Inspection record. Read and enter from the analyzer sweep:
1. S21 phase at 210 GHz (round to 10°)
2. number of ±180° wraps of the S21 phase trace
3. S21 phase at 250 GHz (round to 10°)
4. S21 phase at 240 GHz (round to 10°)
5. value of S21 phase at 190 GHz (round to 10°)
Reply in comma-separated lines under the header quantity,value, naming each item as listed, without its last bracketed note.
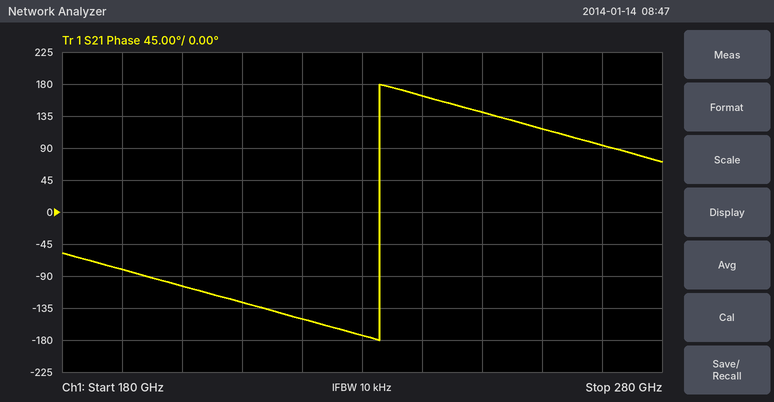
quantity,value
S21 phase at 210 GHz,-130°
number of ±180° wraps of the S21 phase trace,1
S21 phase at 250 GHz,140°
S21 phase at 240 GHz,160°
value of S21 phase at 190 GHz,-80°
